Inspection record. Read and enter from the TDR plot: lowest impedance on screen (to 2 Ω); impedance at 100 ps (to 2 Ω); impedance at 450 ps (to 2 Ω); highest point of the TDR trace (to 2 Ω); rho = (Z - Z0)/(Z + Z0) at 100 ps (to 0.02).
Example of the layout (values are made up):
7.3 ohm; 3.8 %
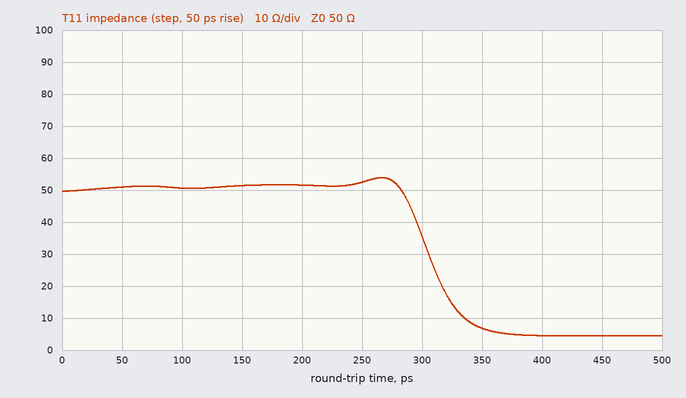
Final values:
4 Ω; 50 Ω; 4 Ω; 54 Ω; 0.00
